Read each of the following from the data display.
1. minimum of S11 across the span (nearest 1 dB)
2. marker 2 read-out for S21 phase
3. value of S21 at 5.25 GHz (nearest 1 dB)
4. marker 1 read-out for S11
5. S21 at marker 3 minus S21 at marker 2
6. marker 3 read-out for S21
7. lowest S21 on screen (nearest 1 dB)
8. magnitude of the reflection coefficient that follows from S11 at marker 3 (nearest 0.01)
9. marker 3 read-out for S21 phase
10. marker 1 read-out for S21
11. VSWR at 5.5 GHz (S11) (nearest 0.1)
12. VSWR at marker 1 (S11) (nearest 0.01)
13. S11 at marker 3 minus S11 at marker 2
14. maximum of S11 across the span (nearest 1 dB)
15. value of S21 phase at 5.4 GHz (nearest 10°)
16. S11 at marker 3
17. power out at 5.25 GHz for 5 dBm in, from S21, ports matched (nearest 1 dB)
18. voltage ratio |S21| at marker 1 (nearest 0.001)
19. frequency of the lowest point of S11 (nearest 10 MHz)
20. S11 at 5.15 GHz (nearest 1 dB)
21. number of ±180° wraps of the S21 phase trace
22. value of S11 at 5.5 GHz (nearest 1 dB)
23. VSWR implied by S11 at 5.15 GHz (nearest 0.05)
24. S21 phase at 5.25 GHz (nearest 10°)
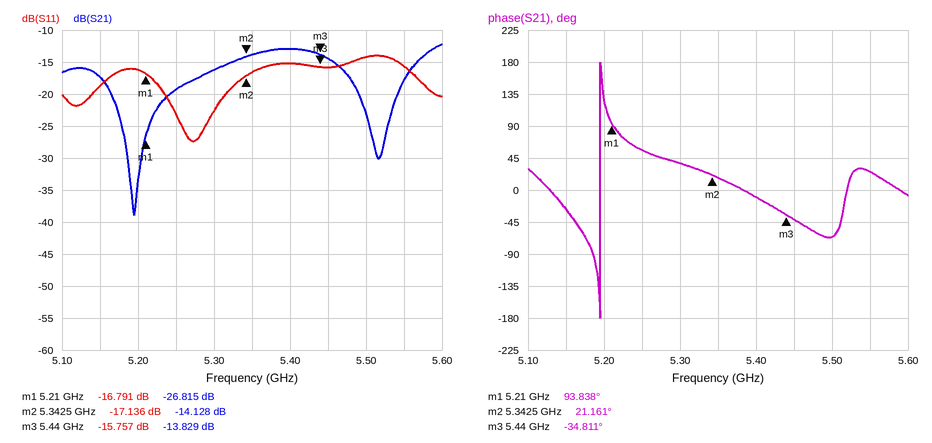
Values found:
-27 dB
21.161°
-19 dB
-16.791 dB
0.299 dB
-13.829 dB
-39 dB
0.16
-34.811°
-26.815 dB
1.5
1.34
1.379 dB
-14 dB
-10°
-15.757 dB
-14 dBm
0.046
5.27 GHz
-19 dB
1
-14 dB
1.25
60°
